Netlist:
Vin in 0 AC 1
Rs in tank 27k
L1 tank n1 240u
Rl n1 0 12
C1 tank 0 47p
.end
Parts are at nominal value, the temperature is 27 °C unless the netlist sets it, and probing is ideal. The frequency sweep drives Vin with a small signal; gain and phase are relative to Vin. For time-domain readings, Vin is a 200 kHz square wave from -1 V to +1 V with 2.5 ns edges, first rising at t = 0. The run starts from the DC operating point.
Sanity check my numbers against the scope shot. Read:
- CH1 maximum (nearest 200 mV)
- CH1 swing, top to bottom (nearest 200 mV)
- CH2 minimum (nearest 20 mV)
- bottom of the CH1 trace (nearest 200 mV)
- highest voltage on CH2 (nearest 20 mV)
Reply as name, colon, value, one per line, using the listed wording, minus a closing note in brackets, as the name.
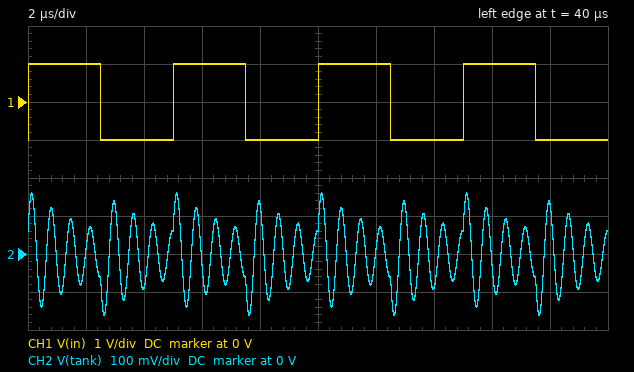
CH1 maximum: 1.0 V
CH1 swing, top to bottom: 2.0 V
CH2 minimum: -160 mV
bottom of the CH1 trace: -1.0 V
highest voltage on CH2: 160 mV
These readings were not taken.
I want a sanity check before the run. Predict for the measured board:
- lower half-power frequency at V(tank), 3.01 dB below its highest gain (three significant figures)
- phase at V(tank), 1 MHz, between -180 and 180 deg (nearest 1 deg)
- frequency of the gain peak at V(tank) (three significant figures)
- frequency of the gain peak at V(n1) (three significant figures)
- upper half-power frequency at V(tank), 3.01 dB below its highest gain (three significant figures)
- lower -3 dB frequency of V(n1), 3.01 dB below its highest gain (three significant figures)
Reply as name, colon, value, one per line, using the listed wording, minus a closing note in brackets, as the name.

lower half-power frequency at V(tank), 3.01 dB below its highest gain: 1.43 MHz
phase at V(tank), 1 MHz, between -180 and 180 deg: 83 deg
frequency of the gain peak at V(tank): 1.50 MHz
frequency of the gain peak at V(n1): 1.50 MHz
upper half-power frequency at V(tank), 3.01 dB below its highest gain: 1.57 MHz
lower -3 dB frequency of V(n1), 3.01 dB below its highest gain: 1.43 MHz
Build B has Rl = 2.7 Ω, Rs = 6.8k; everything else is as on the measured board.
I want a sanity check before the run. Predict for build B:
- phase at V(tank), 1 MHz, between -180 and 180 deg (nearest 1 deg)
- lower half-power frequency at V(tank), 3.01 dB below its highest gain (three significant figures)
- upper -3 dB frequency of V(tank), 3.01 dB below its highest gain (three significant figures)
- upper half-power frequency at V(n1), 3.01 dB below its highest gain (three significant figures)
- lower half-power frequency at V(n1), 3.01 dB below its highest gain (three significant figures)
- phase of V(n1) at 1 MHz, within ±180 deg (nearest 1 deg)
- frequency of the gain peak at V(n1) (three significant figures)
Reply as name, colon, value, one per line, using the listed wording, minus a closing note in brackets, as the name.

phase at V(tank), 1 MHz, between -180 and 180 deg: 68 deg
lower half-power frequency at V(tank), 3.01 dB below its highest gain: 1.27 MHz
upper -3 dB frequency of V(tank), 3.01 dB below its highest gain: 1.77 MHz
upper half-power frequency at V(n1), 3.01 dB below its highest gain: 1.69 MHz
lower half-power frequency at V(n1), 3.01 dB below its highest gain: 1.18 MHz
phase of V(n1) at 1 MHz, within ±180 deg: -22 deg
frequency of the gain peak at V(n1): 1.46 MHz
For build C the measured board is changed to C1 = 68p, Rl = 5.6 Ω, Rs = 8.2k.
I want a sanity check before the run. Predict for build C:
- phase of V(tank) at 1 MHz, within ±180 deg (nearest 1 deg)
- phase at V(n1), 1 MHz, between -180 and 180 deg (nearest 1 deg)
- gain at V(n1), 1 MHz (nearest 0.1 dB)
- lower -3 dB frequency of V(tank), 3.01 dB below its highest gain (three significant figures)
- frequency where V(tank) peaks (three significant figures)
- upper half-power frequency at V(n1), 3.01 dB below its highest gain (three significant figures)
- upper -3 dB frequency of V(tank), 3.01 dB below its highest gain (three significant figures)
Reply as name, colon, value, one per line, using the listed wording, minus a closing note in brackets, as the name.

phase of V(tank) at 1 MHz, within ±180 deg: 62 deg
phase at V(n1), 1 MHz, between -180 and 180 deg: -28 deg
gain at V(n1), 1 MHz: -55.4 dB
lower -3 dB frequency of V(tank), 3.01 dB below its highest gain: 1.11 MHz
frequency where V(tank) peaks: 1.25 MHz
upper half-power frequency at V(n1), 3.01 dB below its highest gain: 1.37 MHz
upper -3 dB frequency of V(tank), 3.01 dB below its highest gain: 1.40 MHz
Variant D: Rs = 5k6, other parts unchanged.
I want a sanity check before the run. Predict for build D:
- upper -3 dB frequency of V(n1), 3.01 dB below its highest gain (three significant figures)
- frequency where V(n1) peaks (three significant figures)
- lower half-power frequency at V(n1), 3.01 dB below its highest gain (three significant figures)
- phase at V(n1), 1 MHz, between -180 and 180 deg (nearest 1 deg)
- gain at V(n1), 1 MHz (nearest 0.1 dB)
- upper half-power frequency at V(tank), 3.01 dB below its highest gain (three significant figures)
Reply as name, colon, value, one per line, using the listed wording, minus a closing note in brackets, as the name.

upper -3 dB frequency of V(n1), 3.01 dB below its highest gain: 1.72 MHz
frequency where V(n1) peaks: 1.44 MHz
lower half-power frequency at V(n1), 3.01 dB below its highest gain: 1.08 MHz
phase at V(n1), 1 MHz, between -180 and 180 deg: -26 deg
gain at V(n1), 1 MHz: -49.2 dB
upper half-power frequency at V(tank), 3.01 dB below its highest gain: 1.84 MHz
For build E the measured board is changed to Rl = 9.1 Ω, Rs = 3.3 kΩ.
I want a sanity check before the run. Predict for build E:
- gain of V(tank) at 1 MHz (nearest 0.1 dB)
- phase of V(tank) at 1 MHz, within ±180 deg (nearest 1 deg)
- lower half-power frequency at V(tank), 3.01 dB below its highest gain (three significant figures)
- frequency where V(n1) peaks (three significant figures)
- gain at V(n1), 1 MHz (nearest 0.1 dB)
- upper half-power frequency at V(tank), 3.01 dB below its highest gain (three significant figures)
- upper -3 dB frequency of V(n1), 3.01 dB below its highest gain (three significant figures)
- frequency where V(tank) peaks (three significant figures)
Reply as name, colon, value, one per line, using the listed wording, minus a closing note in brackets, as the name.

gain of V(tank) at 1 MHz: -4.0 dB
phase of V(tank) at 1 MHz, within ±180 deg: 50 deg
lower half-power frequency at V(tank), 3.01 dB below its highest gain: 1.07 MHz
frequency where V(n1) peaks: 1.31 MHz
gain at V(n1), 1 MHz: -48.4 dB
upper half-power frequency at V(tank), 3.01 dB below its highest gain: 2.10 MHz
upper -3 dB frequency of V(n1), 3.01 dB below its highest gain: 1.78 MHz
frequency where V(tank) peaks: 1.50 MHz
